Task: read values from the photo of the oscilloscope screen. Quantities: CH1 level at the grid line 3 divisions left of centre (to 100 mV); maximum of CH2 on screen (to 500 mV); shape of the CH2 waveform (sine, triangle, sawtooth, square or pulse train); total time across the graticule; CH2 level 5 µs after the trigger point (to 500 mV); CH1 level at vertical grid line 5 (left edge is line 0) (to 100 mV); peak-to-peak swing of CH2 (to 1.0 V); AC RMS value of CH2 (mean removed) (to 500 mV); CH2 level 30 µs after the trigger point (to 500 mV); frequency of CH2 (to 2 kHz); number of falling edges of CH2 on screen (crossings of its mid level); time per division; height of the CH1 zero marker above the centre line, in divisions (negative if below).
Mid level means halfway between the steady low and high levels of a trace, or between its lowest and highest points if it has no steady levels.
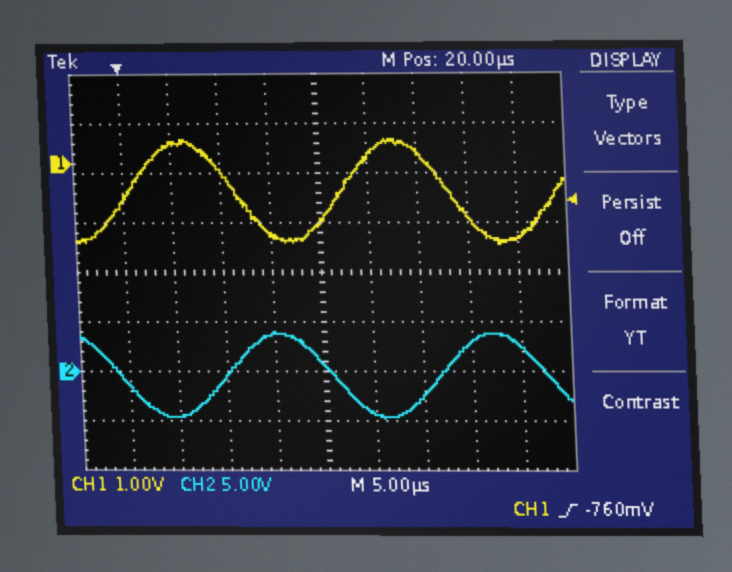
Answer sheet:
400 mV
4.0 V
sine
50 µs
-4.5 V
-1.2 V
9.0 V
3.0 V
-2.5 V
46 kHz
3
5 µs
+2.2 div
